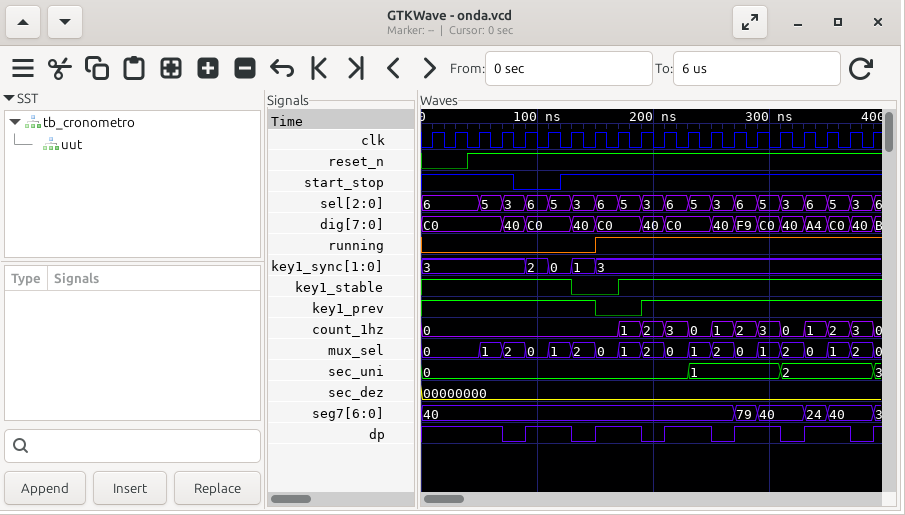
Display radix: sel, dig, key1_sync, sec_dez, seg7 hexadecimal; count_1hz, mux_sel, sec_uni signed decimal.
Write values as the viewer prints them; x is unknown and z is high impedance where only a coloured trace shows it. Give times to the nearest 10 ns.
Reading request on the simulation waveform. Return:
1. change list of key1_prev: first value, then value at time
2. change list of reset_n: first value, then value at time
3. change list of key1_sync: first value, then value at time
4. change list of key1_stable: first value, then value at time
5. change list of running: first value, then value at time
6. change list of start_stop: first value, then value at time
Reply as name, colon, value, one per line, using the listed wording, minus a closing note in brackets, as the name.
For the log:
change list of key1_prev: first value, then value at time: 1, 0 at 150 ns, 1 at 190 ns
change list of reset_n: first value, then value at time: 0, 1 at 40 ns
change list of key1_sync: first value, then value at time: 3, 2 at 90 ns, 0 at 110 ns, 1 at 130 ns, 3 at 150 ns
change list of key1_stable: first value, then value at time: 1, 0 at 130 ns, 1 at 170 ns
change list of running: first value, then value at time: 0, 1 at 150 ns
change list of start_stop: first value, then value at time: 1, 0 at 80 ns, 1 at 120 ns
